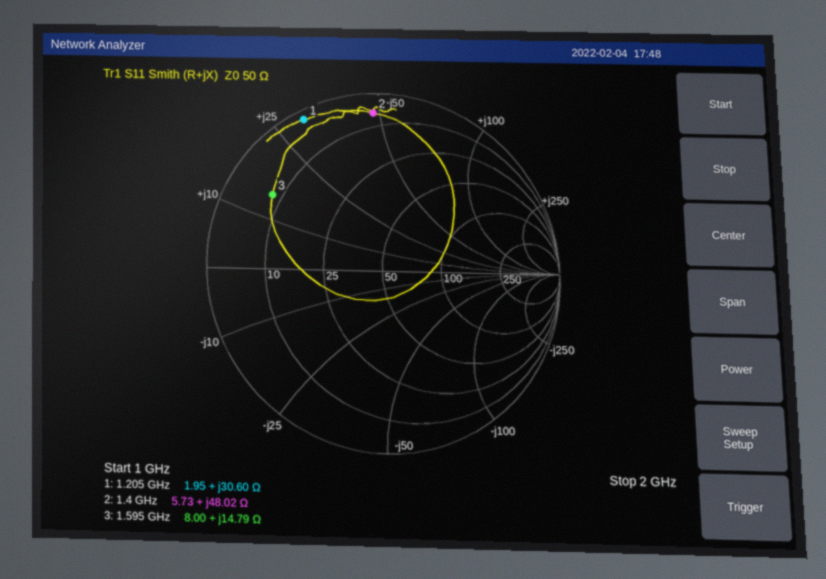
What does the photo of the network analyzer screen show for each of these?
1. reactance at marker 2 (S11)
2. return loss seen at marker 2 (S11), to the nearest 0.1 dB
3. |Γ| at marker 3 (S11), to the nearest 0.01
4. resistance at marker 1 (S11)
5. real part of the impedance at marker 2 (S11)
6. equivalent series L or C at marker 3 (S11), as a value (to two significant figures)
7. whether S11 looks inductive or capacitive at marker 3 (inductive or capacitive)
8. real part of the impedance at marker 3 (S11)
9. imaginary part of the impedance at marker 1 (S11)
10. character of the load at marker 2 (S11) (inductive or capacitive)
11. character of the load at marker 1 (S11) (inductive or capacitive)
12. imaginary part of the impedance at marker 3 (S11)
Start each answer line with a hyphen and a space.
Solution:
- +48.02 Ω
- 1.0 dB
- 0.74
- 1.95 Ω
- 5.73 Ω
- 1.5 nH
- inductive
- 8.00 Ω
- +30.60 Ω
- inductive
- inductive
- +14.79 Ω
